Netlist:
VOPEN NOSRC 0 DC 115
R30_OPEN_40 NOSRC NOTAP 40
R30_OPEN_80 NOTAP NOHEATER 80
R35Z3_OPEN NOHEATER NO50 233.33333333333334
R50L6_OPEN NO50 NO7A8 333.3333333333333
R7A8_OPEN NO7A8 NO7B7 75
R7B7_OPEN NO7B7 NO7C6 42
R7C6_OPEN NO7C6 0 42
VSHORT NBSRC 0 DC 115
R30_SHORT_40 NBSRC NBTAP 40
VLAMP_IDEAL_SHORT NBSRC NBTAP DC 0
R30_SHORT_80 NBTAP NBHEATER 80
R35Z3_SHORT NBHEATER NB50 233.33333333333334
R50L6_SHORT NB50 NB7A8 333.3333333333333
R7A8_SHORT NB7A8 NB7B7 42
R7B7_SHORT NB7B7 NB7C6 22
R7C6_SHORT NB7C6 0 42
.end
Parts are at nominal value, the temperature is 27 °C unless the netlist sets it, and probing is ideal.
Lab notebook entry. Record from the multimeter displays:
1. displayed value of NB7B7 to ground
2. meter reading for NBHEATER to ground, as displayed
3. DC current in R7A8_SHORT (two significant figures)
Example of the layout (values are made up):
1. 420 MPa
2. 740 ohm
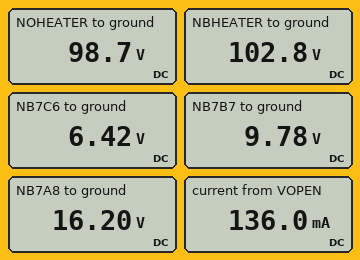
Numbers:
1. 9.78 V
2. 102.8 V
3. 150 mA
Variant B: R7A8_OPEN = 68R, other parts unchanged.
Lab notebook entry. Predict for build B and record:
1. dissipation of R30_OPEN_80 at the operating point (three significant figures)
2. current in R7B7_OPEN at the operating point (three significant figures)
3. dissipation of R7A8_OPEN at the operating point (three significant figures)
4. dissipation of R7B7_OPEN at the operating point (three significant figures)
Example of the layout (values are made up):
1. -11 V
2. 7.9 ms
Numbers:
1. 1.50 W
2. 137 mA
3. 1.28 W
4. 790 mW
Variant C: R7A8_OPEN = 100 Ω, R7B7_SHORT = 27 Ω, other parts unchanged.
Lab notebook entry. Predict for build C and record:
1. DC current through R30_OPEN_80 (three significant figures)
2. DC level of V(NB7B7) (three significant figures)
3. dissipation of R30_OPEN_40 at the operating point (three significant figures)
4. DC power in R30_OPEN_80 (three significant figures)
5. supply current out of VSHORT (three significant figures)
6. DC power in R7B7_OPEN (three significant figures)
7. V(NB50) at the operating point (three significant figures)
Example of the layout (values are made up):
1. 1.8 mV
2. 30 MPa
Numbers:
1. 132 mA
2. 10.5 V
3. 698 mW
4. 1.40 W
5. 152 mA
6. 733 mW
7. 67.4 V
